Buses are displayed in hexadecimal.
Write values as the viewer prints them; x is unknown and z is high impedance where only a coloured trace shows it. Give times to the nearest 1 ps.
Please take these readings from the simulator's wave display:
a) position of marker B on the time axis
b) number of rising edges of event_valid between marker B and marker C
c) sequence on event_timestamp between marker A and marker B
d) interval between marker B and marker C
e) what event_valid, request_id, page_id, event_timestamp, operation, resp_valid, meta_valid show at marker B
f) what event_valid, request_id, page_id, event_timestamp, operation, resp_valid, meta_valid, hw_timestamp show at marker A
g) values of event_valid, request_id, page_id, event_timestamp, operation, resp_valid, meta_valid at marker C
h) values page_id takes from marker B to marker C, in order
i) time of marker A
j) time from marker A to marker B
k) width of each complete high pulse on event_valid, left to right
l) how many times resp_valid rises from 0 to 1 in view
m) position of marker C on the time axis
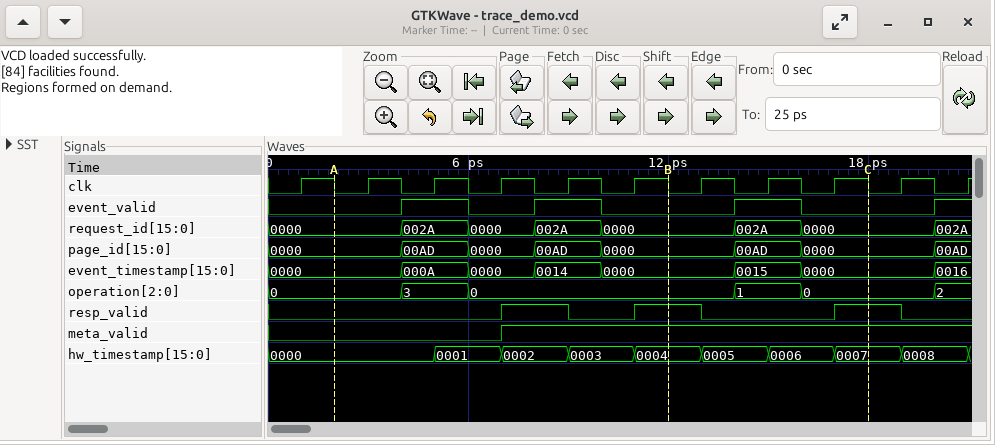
12 ps
1
0000, 000A, 0000, 0014, 0000
6 ps
event_valid=0, request_id=0000, page_id=0000, event_timestamp=0000, operation=0, resp_valid=1, meta_valid=1
event_valid=0, request_id=0000, page_id=0000, event_timestamp=0000, operation=0, resp_valid=0, meta_valid=0, hw_timestamp=0000
event_valid=0, request_id=0000, page_id=0000, event_timestamp=0000, operation=0, resp_valid=1, meta_valid=1
0000, 00AD, 0000
2 ps
10 ps
2 ps, 2 ps, 2 ps
3
18 ps
